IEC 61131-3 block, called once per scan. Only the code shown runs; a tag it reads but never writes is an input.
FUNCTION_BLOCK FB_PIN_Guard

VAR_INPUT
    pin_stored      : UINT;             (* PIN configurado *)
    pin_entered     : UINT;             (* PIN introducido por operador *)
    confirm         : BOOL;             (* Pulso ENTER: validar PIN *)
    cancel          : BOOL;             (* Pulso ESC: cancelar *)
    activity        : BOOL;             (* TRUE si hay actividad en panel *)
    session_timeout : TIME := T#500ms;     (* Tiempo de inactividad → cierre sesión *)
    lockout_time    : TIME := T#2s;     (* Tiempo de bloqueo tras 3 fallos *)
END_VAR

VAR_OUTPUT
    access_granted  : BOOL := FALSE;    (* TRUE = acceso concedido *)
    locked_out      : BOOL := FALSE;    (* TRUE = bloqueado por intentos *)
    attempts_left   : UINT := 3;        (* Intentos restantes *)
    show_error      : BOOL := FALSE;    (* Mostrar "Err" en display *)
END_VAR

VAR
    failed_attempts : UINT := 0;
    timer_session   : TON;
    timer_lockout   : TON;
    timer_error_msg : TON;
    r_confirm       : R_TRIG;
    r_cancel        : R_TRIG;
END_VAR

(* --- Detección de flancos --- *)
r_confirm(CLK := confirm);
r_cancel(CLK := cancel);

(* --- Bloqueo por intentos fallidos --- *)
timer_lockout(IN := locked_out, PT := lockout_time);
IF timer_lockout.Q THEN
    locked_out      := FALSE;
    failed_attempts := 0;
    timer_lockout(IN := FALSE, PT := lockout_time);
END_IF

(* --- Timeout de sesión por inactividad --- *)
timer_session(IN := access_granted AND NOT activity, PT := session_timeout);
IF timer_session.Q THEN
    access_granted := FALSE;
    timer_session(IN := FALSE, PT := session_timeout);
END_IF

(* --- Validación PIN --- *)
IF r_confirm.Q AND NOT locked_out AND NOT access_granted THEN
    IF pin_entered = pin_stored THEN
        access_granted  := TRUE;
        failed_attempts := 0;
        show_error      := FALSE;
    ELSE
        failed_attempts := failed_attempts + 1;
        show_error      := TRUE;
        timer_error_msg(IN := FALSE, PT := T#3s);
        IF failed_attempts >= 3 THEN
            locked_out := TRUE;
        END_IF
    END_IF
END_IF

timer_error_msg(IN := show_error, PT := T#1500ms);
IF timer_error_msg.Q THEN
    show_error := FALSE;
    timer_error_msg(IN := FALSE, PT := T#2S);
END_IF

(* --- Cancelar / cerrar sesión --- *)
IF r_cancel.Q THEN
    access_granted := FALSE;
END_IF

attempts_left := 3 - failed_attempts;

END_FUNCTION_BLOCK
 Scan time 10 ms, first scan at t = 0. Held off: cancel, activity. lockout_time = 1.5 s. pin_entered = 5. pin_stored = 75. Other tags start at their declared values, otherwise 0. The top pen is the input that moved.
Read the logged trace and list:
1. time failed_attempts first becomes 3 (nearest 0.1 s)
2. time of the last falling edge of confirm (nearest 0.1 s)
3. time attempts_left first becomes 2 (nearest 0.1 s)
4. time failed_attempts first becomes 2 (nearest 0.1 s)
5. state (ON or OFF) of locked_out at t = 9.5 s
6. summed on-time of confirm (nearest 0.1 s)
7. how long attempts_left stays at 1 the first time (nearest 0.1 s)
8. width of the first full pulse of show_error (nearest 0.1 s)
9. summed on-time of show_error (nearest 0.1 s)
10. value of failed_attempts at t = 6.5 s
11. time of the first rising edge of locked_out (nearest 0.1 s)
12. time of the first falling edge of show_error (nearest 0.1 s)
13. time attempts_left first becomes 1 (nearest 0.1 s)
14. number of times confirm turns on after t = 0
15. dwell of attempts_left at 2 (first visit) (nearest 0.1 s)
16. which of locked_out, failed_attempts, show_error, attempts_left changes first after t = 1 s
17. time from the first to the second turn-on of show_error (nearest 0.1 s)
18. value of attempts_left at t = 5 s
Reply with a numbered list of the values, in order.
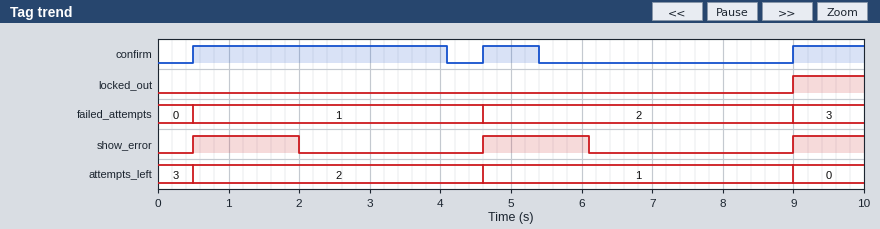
1. 9.0 s
2. 5.4 s
3. 0.5 s
4. 4.6 s
5. ON
6. 5.4 s
7. 4.4 s
8. 1.5 s
9. 4.0 s
10. 2
11. 9.0 s
12. 2.0 s
13. 4.6 s
14. 3
15. 4.1 s
16. show_error
17. 4.1 s
18. 1
